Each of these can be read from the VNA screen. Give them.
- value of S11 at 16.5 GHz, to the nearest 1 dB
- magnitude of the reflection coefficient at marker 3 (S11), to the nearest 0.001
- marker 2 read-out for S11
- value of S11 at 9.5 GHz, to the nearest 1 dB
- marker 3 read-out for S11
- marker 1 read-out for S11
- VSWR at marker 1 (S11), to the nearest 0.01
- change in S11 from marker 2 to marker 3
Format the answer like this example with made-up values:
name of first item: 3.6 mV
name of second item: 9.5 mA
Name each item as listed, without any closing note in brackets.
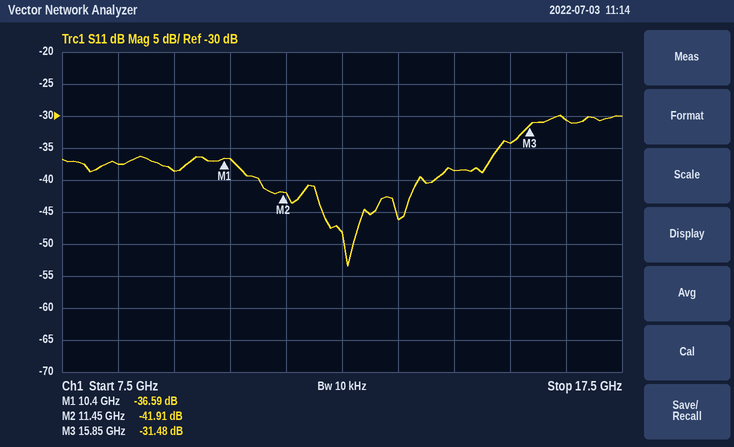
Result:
value of S11 at 16.5 GHz, to the nearest 1 dB: -31 dB
magnitude of the reflection coefficient at marker 3 (S11), to the nearest 0.001: 0.027
marker 2 read-out for S11: -41.91 dB
value of S11 at 9.5 GHz, to the nearest 1 dB: -39 dB
marker 3 read-out for S11: -31.48 dB
marker 1 read-out for S11: -36.59 dB
VSWR at marker 1 (S11), to the nearest 0.01: 1.03
change in S11 from marker 2 to marker 3: 10.43 dB
